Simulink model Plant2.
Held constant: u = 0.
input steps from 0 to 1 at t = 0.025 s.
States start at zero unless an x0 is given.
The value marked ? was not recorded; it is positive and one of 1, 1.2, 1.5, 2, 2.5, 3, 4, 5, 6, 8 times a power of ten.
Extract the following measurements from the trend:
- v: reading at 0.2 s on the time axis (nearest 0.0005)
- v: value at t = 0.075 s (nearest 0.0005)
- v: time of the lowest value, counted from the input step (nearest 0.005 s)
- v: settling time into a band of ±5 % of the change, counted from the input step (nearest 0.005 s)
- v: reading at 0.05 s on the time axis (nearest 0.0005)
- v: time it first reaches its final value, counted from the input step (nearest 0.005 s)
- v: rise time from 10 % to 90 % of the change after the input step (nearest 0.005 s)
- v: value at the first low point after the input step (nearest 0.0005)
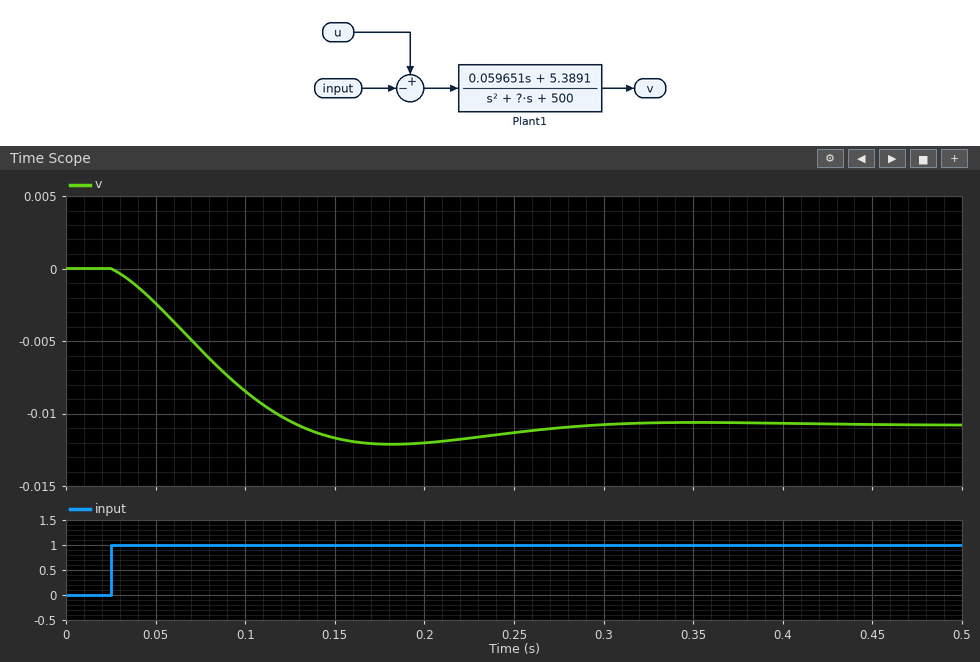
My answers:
-0.0120
-0.0055
0.155 s
0.225 s
-0.0025
0.105 s
0.075 s
-0.0120
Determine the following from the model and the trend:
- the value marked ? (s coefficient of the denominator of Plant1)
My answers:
25
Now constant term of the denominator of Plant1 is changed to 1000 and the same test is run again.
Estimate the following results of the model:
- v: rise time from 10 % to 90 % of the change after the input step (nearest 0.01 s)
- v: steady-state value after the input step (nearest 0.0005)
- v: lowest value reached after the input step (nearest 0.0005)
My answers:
0.04 s
-0.0055
-0.0070
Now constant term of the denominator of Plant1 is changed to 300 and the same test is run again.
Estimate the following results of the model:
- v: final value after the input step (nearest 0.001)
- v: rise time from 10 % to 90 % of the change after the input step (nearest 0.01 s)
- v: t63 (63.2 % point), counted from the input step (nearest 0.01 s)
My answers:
-0.018
0.12 s
0.09 s
